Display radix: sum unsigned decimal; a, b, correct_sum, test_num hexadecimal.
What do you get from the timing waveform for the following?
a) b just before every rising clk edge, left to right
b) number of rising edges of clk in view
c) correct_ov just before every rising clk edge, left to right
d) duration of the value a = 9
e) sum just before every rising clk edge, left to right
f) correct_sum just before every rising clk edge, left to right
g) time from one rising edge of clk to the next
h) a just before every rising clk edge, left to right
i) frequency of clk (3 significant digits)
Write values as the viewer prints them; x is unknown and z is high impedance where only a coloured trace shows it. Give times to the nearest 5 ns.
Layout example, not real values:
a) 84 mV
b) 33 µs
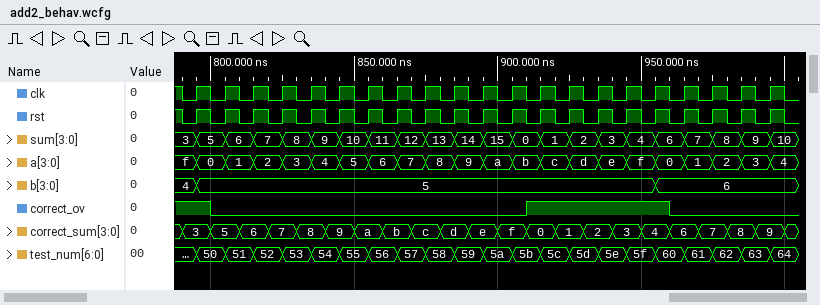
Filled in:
a) 4, 5, 5, 5, 5, 5, 5, 5, 5, 5, 5, 5, 5, 5, 5, 5, 5, 6, 6, 6, 6
b) 21
c) 1 0 0 0 0 0 0 0 0 0 0 0 1 1 1 1 1 0 0 0 0
d) 10 ns
e) 3, 5, 6, 7, 8, 9, 10, 11, 12, 13, 14, 15, 0, 1, 2, 3, 4, 6, 7, 8, 9
f) 3, 5, 6, 7, 8, 9, a, b, c, d, e, f, 0, 1, 2, 3, 4, 6, 7, 8, 9
g) 10 ns
h) f, 0, 1, 2, 3, 4, 5, 6, 7, 8, 9, a, b, c, d, e, f, 0, 1, 2, 3
i) 100 MHz
